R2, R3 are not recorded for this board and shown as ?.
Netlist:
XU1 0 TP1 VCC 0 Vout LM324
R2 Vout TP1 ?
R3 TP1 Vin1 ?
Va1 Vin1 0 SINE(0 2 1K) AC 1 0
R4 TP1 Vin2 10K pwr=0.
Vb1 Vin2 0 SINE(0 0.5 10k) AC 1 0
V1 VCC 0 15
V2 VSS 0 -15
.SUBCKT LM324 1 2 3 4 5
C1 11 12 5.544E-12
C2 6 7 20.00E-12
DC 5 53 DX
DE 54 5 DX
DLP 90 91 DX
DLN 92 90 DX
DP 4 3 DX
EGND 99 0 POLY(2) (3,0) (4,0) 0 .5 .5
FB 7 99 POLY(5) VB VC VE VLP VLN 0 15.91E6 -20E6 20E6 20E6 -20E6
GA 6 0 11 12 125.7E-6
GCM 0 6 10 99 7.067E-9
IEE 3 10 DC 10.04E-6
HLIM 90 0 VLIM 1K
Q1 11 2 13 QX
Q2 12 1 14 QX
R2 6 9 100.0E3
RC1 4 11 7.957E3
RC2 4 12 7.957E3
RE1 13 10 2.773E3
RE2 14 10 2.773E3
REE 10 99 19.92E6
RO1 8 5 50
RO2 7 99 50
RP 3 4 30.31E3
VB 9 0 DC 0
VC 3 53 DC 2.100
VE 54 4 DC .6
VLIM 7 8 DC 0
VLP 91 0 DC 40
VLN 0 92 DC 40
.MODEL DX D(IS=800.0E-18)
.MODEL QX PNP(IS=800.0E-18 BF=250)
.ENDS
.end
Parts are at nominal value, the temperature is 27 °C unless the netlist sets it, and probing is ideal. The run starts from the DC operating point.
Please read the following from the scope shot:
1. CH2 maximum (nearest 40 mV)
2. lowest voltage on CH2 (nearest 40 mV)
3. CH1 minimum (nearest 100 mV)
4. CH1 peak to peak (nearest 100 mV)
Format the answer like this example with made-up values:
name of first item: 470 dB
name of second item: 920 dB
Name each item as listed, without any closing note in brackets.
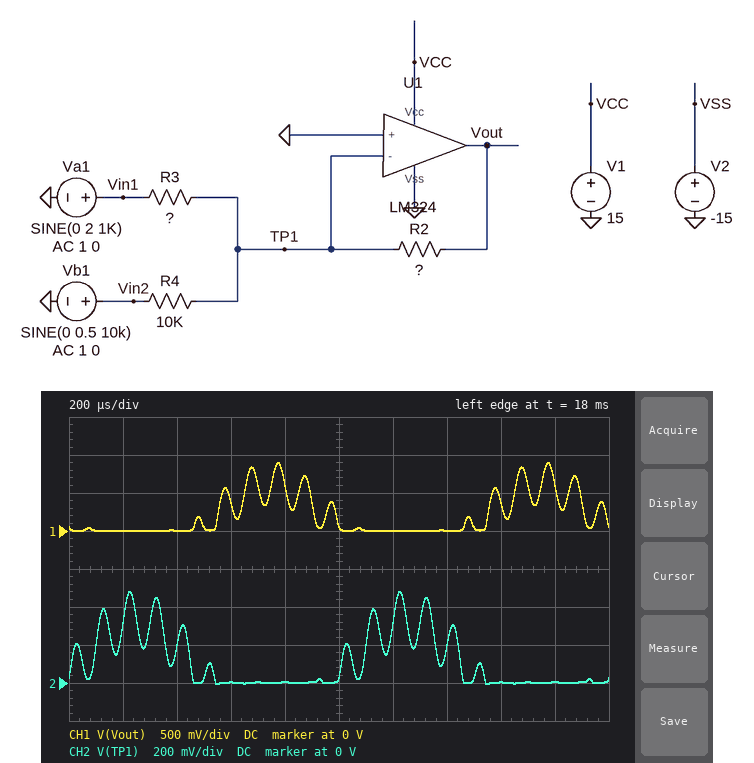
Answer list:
CH2 maximum: 480 mV
lowest voltage on CH2: 0 V
CH1 minimum: 0 V
CH1 peak to peak: 900 mV
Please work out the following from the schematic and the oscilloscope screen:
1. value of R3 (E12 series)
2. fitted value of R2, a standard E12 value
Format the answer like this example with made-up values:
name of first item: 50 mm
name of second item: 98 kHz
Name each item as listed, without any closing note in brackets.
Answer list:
value of R3: 18 kΩ
fitted value of R2, a standard E12 value: 5.6 kΩ
